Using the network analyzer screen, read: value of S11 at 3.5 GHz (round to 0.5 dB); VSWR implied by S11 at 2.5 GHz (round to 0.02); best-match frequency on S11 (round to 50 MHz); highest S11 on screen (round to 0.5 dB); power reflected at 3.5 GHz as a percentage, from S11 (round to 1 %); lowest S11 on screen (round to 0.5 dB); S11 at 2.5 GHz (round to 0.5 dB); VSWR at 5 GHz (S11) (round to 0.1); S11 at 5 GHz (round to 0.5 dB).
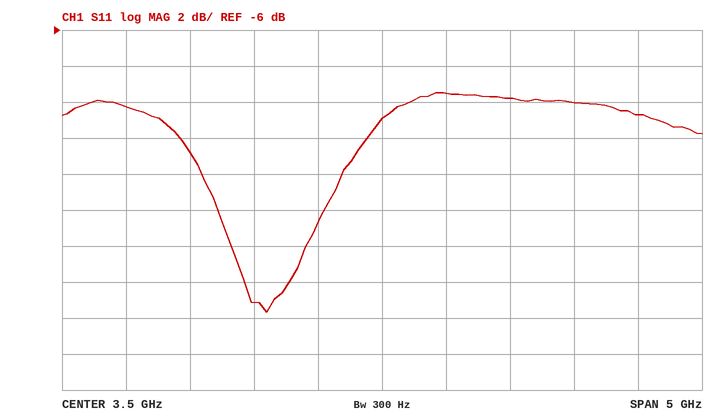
-11.0 dB
1.20
2.60 GHz
-9.5 dB
8 %
-21.5 dB
-21.0 dB
1.9
-10.0 dB
